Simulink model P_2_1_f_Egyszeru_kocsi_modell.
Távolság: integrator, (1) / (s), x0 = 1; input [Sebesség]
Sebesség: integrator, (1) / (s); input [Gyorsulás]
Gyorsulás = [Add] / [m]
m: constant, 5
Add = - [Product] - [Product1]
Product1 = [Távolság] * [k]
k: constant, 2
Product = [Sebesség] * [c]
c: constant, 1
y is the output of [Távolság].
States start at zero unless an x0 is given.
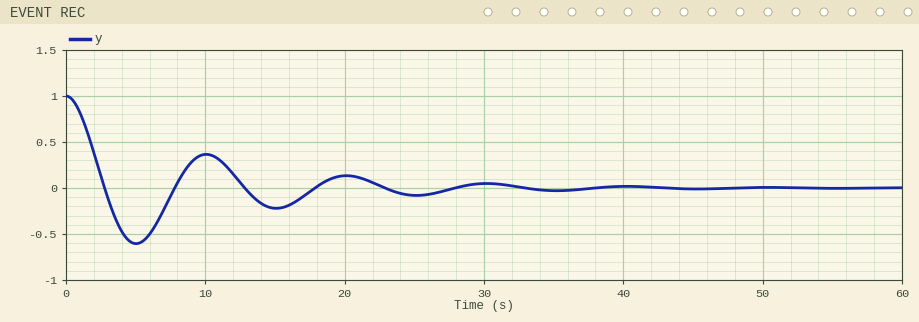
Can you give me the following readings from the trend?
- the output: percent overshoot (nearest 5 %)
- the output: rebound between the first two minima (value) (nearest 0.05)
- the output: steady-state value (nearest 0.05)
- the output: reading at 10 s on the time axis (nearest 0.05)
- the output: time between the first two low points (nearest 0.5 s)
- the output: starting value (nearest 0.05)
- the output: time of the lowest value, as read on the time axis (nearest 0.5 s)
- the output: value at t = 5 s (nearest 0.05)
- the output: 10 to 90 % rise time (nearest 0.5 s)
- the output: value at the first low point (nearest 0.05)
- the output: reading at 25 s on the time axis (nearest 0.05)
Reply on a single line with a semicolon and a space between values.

60 %; 0.35; 0.00; 0.35; 10.0 s; 1.00; 5.0 s; -0.60; 2.0 s; -0.60; -0.10
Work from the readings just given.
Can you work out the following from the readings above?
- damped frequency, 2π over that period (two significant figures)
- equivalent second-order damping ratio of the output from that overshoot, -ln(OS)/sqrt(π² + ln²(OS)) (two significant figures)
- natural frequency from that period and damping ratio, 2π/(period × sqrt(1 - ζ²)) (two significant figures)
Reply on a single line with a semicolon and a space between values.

0.63 rad/s; 0.16; 0.64 rad/s
